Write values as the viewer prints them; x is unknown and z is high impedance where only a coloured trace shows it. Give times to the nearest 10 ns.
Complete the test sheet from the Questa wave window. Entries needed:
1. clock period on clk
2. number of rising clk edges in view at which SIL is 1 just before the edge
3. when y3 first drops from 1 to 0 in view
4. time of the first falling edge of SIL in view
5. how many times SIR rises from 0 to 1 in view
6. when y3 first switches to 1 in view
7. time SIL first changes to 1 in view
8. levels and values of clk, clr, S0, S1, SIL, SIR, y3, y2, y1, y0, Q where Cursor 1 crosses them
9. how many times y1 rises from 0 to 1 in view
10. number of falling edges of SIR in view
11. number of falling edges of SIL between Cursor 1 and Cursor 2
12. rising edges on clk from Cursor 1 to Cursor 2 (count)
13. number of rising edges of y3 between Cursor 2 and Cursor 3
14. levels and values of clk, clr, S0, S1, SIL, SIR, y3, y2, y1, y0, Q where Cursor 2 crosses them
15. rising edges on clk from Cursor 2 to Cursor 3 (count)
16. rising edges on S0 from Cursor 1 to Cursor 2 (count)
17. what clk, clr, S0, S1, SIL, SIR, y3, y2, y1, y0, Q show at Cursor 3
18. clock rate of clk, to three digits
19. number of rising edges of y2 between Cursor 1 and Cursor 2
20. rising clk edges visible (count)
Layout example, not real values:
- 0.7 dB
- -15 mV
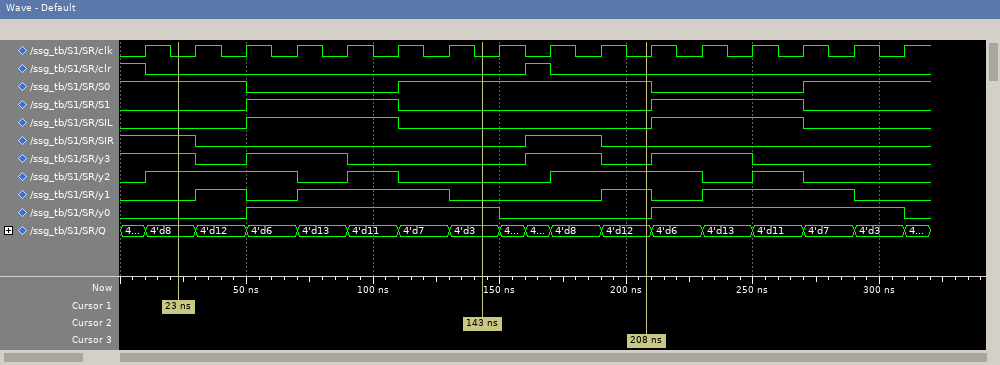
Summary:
- 20 ns
- 6
- 30 ns
- 110 ns
- 1
- 50 ns
- 50 ns
- clk=0, clr=0, S0=1, S1=0, SIL=0, SIR=1, y3=1, y2=1, y1=0, y0=0, Q=4'd8
- 4
- 2
- 1
- 6
- 1
- clk=0, clr=0, S0=1, S1=0, SIL=0, SIR=0, y3=0, y2=0, y1=0, y0=1, Q=4'd3
- 3
- 1
- clk=0, clr=0, S0=1, S1=0, SIL=0, SIR=0, y3=0, y2=1, y1=1, y0=0, Q=4'd12
- 50.0 MHz
- 1
- 16
